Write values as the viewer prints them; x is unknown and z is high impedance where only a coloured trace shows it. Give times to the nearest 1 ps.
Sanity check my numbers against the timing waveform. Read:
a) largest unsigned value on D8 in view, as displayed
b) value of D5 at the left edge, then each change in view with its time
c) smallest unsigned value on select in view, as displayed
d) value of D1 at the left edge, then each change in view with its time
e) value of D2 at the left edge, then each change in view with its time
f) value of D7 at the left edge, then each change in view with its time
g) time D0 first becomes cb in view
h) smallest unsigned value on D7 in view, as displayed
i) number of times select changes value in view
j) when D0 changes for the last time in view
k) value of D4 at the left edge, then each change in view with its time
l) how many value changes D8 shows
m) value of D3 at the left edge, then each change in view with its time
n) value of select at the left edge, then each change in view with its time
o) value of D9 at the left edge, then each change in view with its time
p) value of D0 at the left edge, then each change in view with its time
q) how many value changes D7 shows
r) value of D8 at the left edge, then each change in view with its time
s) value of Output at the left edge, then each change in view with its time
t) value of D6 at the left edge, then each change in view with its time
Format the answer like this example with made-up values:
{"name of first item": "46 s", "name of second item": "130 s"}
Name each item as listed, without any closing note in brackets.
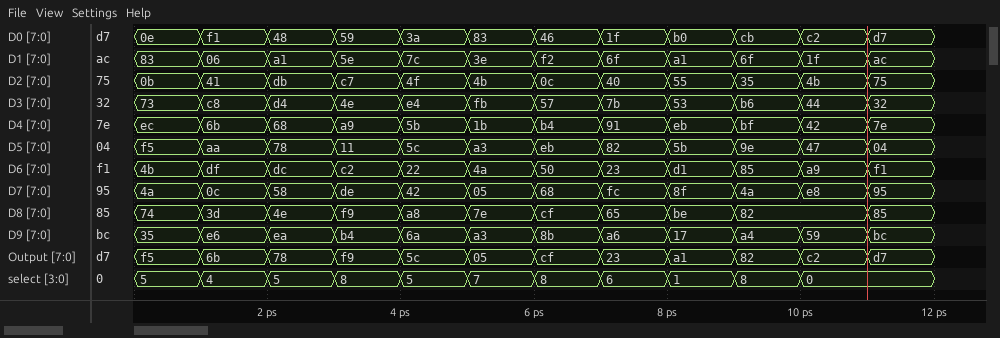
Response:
{"largest unsigned value on D8 in view, as displayed": "f9", "value of D5 at the left edge, then each change in view with its time": "f5, aa at 1 ps, 78 at 2 ps, 11 at 3 ps, 5c at 4 ps, a3 at 5 ps, eb at 6 ps, 82 at 7 ps, 5b at 8 ps, 9e at 9 ps, 47 at 10 ps, 04 at 11 ps", "smallest unsigned value on select in view, as displayed": "0", "value of D1 at the left edge, then each change in view with its time": "83, 06 at 1 ps, a1 at 2 ps, 5e at 3 ps, 7c at 4 ps, 3e at 5 ps, f2 at 6 ps, 6f at 7 ps, a1 at 8 ps, 6f at 9 ps, 1f at 10 ps, ac at 11 ps", "value of D2 at the left edge, then each change in view with its time": "0b, 41 at 1 ps, db at 2 ps, c7 at 3 ps, 4f at 4 ps, 4b at 5 ps, 0c at 6 ps, 40 at 7 ps, 55 at 8 ps, 35 at 9 ps, 4b at 10 ps, 75 at 11 ps", "value of D7 at the left edge, then each change in view with its time": "4a, 0c at 1 ps, 58 at 2 ps, de at 3 ps, 42 at 4 ps, 05 at 5 ps, 68 at 6 ps, fc at 7 ps, 8f at 8 ps, 4a at 9 ps, e8 at 10 ps, 95 at 11 ps", "time D0 first becomes cb in view": "9 ps", "smallest unsigned value on D7 in view, as displayed": "05", "number of times select changes value in view": "10", "when D0 changes for the last time in view": "11 ps", "value of D4 at the left edge, then each change in view with its time": "ec, 6b at 1 ps, 68 at 2 ps, a9 at 3 ps, 5b at 4 ps, 1b at 5 ps, b4 at 6 ps, 91 at 7 ps, eb at 8 ps, bf at 9 ps, 42 at 10 ps, 7e at 11 ps", "how many value changes D8 shows": "10", "value of D3 at the left edge, then each change in view with its time": "73, c8 at 1 ps, d4 at 2 ps, 4e at 3 ps, e4 at 4 ps, fb at 5 ps, 57 at 6 ps, 7b at 7 ps, 53 at 8 ps, b6 at 9 ps, 44 at 10 ps, 32 at 11 ps", "value of select at the left edge, then each change in view with its time": "5, 4 at 1 ps, 5 at 2 ps, 8 at 3 ps, 5 at 4 ps, 7 at 5 ps, 8 at 6 ps, 6 at 7 ps, 1 at 8 ps, 8 at 9 ps, 0 at 10 ps", "value of D9 at the left edge, then each change in view with its time": "35, e6 at 1 ps, ea at 2 ps, b4 at 3 ps, 6a at 4 ps, a3 at 5 ps, 8b at 6 ps, a6 at 7 ps, 17 at 8 ps, a4 at 9 ps, 59 at 10 ps, bc at 11 ps", "value of D0 at the left edge, then each change in view with its time": "0e, f1 at 1 ps, 48 at 2 ps, 59 at 3 ps, 3a at 4 ps, 83 at 5 ps, 46 at 6 ps, 1f at 7 ps, b0 at 8 ps, cb at 9 ps, c2 at 10 ps, d7 at 11 ps", "how many value changes D7 shows": "11", "value of D8 at the left edge, then each change in view with its time": "74, 3d at 1 ps, 4e at 2 ps, f9 at 3 ps, a8 at 4 ps, 7e at 5 ps, cf at 6 ps, 65 at 7 ps, be at 8 ps, 82 at 9 ps, 85 at 11 ps", "value of Output at the left edge, then each change in view with its time": "f5, 6b at 1 ps, 78 at 2 ps, f9 at 3 ps, 5c at 4 ps, 05 at 5 ps, cf at 6 ps, 23 at 7 ps, a1 at 8 ps, 82 at 9 ps, c2 at 10 ps, d7 at 11 ps", "value of D6 at the left edge, then each change in view with its time": "4b, df at 1 ps, dc at 2 ps, c2 at 3 ps, 22 at 4 ps, 4a at 5 ps, 50 at 6 ps, 23 at 7 ps, d1 at 8 ps, 85 at 9 ps, a9 at 10 ps, f1 at 11 ps"}
